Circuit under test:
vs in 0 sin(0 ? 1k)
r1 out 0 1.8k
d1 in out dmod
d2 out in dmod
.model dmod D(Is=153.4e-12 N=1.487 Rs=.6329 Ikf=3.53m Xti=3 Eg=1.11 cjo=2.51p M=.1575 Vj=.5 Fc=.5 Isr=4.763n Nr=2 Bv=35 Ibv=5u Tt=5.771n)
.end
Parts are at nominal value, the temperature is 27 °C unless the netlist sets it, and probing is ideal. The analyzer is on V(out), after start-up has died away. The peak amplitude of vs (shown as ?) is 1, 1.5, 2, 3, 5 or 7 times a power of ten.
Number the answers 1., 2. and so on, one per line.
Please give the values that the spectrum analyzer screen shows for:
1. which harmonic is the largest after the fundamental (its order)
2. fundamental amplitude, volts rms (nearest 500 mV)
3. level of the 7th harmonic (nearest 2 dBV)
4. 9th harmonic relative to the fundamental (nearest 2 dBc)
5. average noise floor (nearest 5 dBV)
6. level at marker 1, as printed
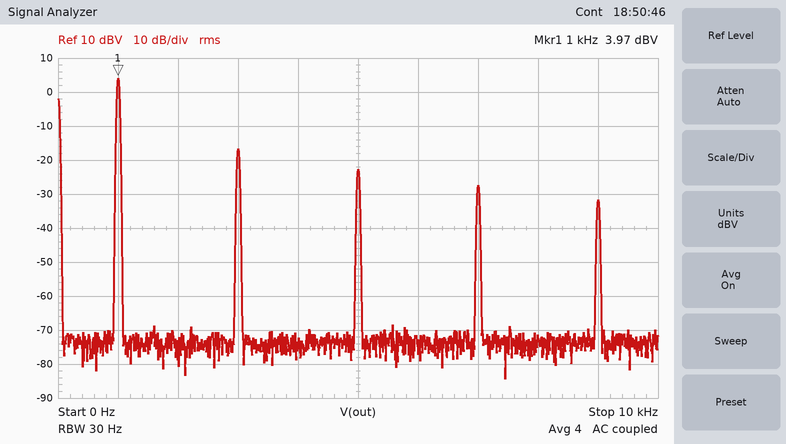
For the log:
1. 3
2. 1.5 V
3. -28 dBV
4. -36 dBc
5. -75 dBV
6. 3.97 dBV
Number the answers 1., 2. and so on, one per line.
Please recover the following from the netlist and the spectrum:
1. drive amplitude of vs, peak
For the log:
1. 3 V
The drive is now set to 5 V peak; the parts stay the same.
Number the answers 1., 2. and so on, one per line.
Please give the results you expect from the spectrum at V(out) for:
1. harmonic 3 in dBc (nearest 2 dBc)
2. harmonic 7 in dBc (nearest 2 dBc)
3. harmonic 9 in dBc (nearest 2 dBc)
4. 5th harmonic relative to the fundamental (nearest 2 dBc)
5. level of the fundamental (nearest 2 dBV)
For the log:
1. -26 dBc
2. -34 dBc
3. -38 dBc
4. -30 dBc
5. 10 dBV
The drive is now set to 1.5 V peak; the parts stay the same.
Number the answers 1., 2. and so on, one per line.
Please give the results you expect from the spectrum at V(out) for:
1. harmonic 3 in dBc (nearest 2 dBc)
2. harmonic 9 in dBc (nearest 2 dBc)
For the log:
1. -14 dBc
2. -46 dBc
